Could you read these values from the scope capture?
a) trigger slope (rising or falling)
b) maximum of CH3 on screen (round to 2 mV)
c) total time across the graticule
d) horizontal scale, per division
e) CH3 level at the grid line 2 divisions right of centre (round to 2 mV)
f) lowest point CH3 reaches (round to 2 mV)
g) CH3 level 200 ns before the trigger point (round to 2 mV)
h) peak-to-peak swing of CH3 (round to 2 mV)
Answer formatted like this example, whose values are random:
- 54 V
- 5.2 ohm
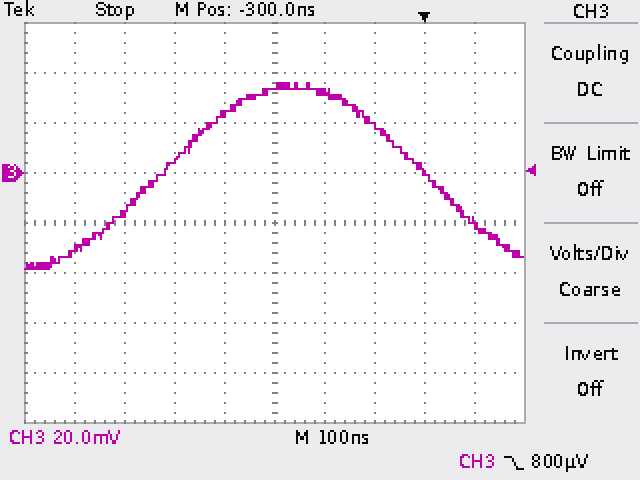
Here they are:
- falling
- 36 mV
- 1 µs
- 100 ns
- 18 mV
- -38 mV
- 32 mV
- 74 mV
